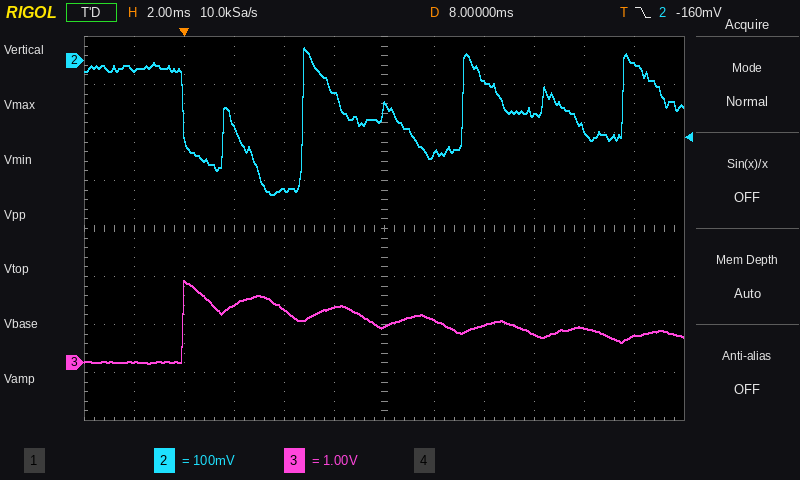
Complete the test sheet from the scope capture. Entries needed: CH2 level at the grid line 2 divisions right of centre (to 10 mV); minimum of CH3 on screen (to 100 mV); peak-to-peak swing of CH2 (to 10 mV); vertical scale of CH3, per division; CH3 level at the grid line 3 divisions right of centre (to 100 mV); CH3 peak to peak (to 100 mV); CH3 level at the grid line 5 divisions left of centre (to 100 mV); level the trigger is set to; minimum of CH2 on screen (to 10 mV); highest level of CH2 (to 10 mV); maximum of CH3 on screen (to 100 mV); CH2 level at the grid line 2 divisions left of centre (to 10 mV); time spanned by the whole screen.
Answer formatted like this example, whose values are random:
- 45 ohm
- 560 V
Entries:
- -40 mV
- 0.0 V
- 310 mV
- 1 V
- 600 mV
- 1.7 V
- 0.0 V
- -160 mV
- -280 mV
- 30 mV
- 1.7 V
- -270 mV
- 24 ms
